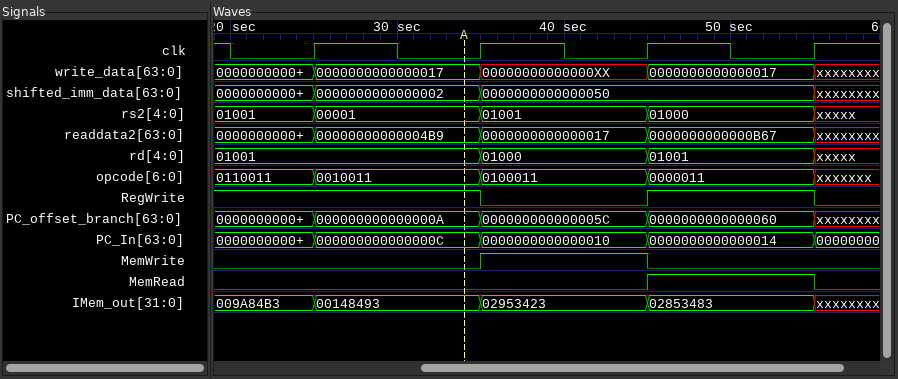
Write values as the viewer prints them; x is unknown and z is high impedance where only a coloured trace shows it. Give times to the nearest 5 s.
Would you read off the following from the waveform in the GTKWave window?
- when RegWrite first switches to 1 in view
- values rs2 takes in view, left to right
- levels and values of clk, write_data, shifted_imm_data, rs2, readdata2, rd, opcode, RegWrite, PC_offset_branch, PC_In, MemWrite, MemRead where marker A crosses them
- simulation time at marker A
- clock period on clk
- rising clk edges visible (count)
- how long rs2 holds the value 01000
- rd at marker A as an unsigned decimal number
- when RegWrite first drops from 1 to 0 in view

45 s
01001, 00001, 01001, 01000, xxxxx
clk=0, write_data=0000000000000017, shifted_imm_data=0000000000000002, rs2=00001, readdata2=00000000000004B9, rd=01001, opcode=0010011, RegWrite=1, PC_offset_branch=000000000000000A, PC_In=000000000000000C, MemWrite=0, MemRead=0
35 s
10 s
4
10 s
9
35 s
